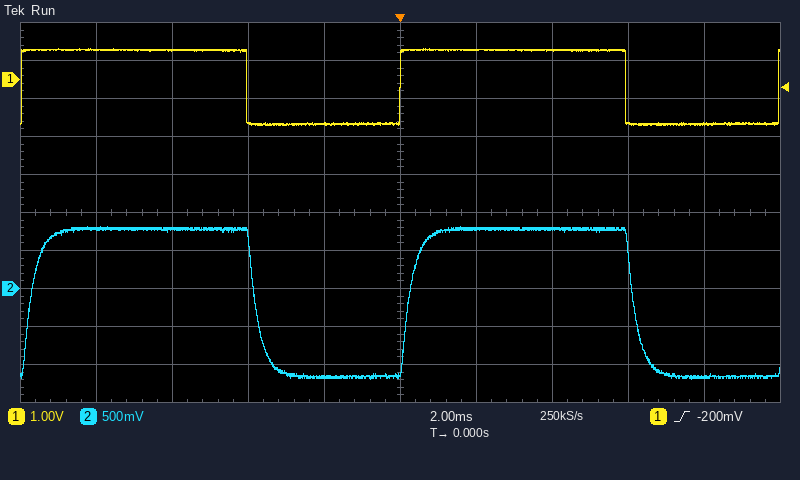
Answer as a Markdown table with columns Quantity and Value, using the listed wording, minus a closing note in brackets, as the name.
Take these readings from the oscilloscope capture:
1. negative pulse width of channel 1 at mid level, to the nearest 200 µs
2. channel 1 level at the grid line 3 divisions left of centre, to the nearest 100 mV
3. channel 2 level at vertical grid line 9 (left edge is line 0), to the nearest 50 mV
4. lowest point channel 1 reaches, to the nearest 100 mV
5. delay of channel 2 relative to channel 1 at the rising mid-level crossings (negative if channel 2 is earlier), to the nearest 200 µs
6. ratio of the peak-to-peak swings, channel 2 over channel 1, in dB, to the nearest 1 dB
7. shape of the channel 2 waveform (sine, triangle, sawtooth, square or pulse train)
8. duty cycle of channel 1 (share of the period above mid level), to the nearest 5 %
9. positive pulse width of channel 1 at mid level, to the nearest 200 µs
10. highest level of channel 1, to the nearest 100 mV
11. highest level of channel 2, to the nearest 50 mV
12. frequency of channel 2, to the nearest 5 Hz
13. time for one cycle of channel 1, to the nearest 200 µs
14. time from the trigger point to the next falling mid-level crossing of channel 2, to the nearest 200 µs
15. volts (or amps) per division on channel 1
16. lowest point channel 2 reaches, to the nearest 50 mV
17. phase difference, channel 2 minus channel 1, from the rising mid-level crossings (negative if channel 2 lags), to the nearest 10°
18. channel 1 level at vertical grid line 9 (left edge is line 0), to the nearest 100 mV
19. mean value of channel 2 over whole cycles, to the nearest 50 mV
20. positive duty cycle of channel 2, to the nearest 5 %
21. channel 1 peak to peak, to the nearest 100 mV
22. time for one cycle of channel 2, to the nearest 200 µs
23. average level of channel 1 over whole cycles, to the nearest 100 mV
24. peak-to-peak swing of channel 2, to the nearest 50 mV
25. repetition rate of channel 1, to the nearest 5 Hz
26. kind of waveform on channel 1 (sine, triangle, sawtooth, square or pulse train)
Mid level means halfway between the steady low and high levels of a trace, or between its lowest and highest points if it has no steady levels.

| Quantity | Value |
|---|---|
| negative pulse width of channel 1 at mid level, to the nearest 200 µs | 4.0 ms |
| channel 1 level at the grid line 3 divisions left of centre, to the nearest 100 mV | 800 mV |
| channel 2 level at vertical grid line 9 (left edge is line 0), to the nearest 50 mV | -1.15 V |
| lowest point channel 1 reaches, to the nearest 100 mV | -1.2 V |
| delay of channel 2 relative to channel 1 at the rising mid-level crossings (negative if channel 2 is earlier), to the nearest 200 µs | +200 µs |
| ratio of the peak-to-peak swings, channel 2 over channel 1, in dB, to the nearest 1 dB | 0 dB |
| shape of the channel 2 waveform | pulse train |
| duty cycle of channel 1 (share of the period above mid level), to the nearest 5 % | 60 % |
| positive pulse width of channel 1 at mid level, to the nearest 200 µs | 6.0 ms |
| highest level of channel 1, to the nearest 100 mV | 800 mV |
| highest level of channel 2, to the nearest 50 mV | 800 mV |
| frequency of channel 2, to the nearest 5 Hz | 100 Hz |
| time for one cycle of channel 1, to the nearest 200 µs | 10.0 ms |
| time from the trigger point to the next falling mid-level crossing of channel 2, to the nearest 200 µs | 6.2 ms |
| volts (or amps) per division on channel 1 | 1 V |
| lowest point channel 2 reaches, to the nearest 50 mV | -1.20 V |
| phase difference, channel 2 minus channel 1, from the rising mid-level crossings (negative if channel 2 lags), to the nearest 10° | -10° |
| channel 1 level at vertical grid line 9 (left edge is line 0), to the nearest 100 mV | -1.2 V |
| mean value of channel 2 over whole cycles, to the nearest 50 mV | 0 mV |
| positive duty cycle of channel 2, to the nearest 5 % | 60 % |
| channel 1 peak to peak, to the nearest 100 mV | 2.0 V |
| time for one cycle of channel 2, to the nearest 200 µs | 10.0 ms |
| average level of channel 1 over whole cycles, to the nearest 100 mV | 0.0 V |
| peak-to-peak swing of channel 2, to the nearest 50 mV | 2.00 V |
| repetition rate of channel 1, to the nearest 5 Hz | 100 Hz |
| kind of waveform on channel 1 | pulse train |
